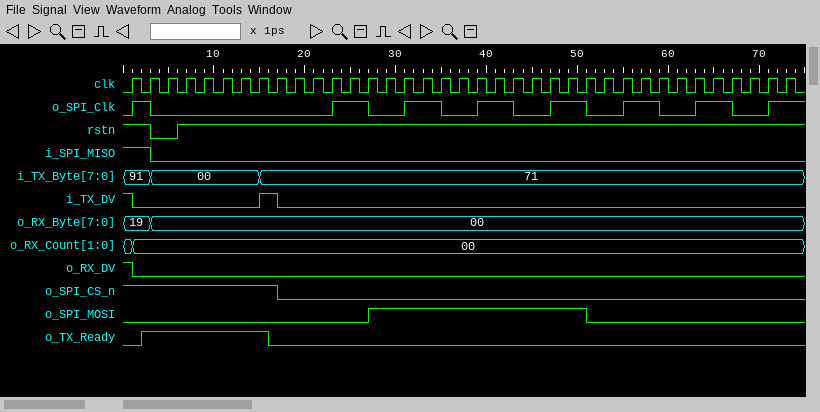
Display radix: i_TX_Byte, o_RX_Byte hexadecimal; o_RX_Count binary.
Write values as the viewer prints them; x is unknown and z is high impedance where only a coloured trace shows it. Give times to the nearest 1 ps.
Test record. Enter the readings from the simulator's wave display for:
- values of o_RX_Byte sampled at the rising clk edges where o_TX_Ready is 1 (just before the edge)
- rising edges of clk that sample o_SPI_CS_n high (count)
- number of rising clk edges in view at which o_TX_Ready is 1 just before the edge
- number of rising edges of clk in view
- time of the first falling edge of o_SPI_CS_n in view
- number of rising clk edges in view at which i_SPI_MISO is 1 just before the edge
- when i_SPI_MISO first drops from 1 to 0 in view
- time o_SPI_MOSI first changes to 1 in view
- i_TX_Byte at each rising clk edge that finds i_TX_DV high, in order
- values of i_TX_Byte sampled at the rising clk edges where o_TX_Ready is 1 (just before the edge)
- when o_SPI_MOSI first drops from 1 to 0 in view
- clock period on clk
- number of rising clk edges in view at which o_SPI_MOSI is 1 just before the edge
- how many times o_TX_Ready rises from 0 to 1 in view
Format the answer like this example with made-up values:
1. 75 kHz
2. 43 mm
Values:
1. 19, 00, 00, 00, 00, 00, 00
2. 9
3. 7
4. 37
5. 17 ps
6. 2
7. 3 ps
8. 27 ps
9. 91, 71
10. 91, 00, 00, 00, 00, 00, 00
11. 51 ps
12. 2 ps
13. 12
14. 1
